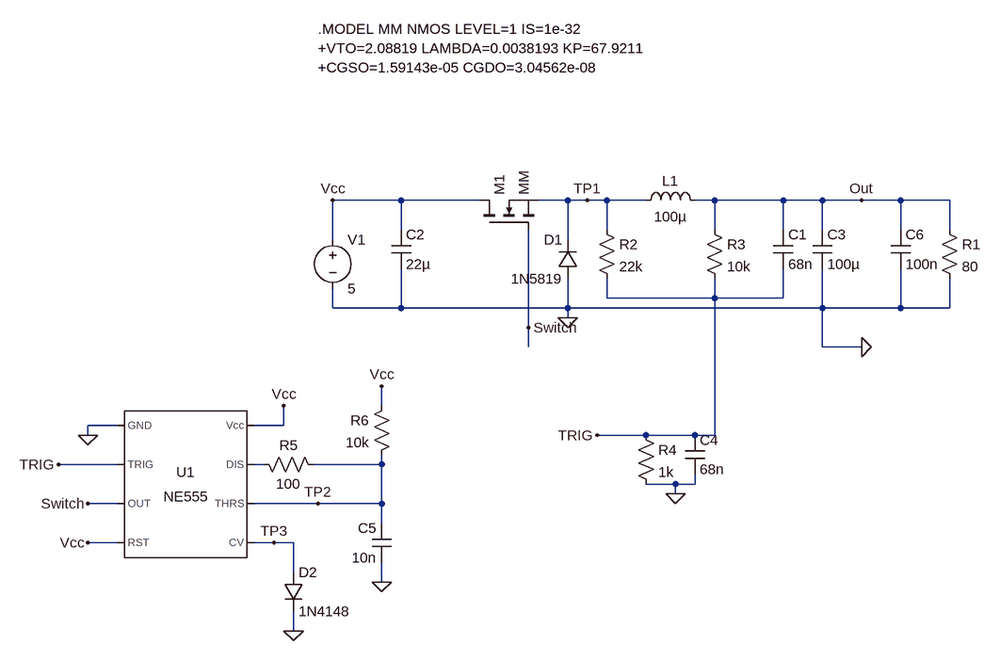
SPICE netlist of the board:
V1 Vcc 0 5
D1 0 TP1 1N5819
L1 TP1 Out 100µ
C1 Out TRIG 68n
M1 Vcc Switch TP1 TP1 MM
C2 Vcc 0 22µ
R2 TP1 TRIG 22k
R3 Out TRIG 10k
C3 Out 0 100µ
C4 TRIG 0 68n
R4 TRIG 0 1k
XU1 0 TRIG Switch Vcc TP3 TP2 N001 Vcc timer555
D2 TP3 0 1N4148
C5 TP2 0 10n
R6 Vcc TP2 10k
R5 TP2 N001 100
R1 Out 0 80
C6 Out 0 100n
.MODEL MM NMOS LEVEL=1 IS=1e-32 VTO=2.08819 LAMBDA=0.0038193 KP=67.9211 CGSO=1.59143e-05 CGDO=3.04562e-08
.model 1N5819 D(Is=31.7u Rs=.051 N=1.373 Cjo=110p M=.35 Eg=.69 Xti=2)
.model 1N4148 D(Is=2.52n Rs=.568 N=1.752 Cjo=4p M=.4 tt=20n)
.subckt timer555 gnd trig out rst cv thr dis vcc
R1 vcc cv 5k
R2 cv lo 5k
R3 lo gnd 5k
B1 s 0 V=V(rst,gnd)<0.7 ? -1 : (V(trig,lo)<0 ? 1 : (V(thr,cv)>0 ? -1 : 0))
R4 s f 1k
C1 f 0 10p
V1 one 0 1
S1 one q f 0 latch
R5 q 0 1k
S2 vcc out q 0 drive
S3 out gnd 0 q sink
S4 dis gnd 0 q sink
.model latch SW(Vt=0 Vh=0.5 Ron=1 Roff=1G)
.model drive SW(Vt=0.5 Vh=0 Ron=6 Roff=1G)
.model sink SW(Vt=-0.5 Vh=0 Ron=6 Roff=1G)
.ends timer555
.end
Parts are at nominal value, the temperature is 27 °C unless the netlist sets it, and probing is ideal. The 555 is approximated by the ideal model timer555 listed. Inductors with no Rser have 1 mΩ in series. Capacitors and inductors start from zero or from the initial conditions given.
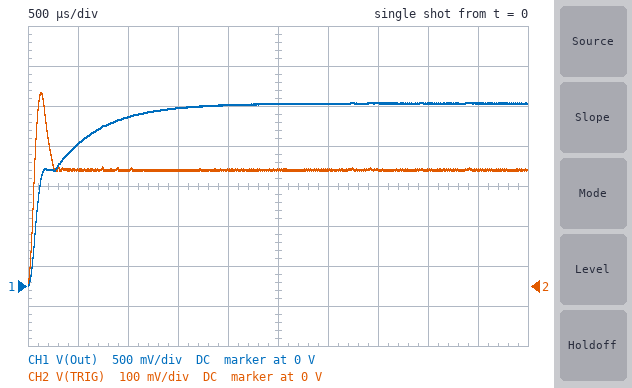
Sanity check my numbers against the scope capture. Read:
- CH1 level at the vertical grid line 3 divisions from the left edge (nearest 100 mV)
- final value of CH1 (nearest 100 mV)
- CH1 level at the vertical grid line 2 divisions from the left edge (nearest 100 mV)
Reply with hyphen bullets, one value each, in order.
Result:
- 2.2 V
- 2.3 V
- 2.1 V
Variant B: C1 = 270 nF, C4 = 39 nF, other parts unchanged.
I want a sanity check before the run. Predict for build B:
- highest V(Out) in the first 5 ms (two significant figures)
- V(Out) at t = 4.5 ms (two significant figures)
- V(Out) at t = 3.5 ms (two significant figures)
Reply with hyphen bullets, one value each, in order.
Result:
- 2.2 V
- 2.1 V
- 2.0 V
